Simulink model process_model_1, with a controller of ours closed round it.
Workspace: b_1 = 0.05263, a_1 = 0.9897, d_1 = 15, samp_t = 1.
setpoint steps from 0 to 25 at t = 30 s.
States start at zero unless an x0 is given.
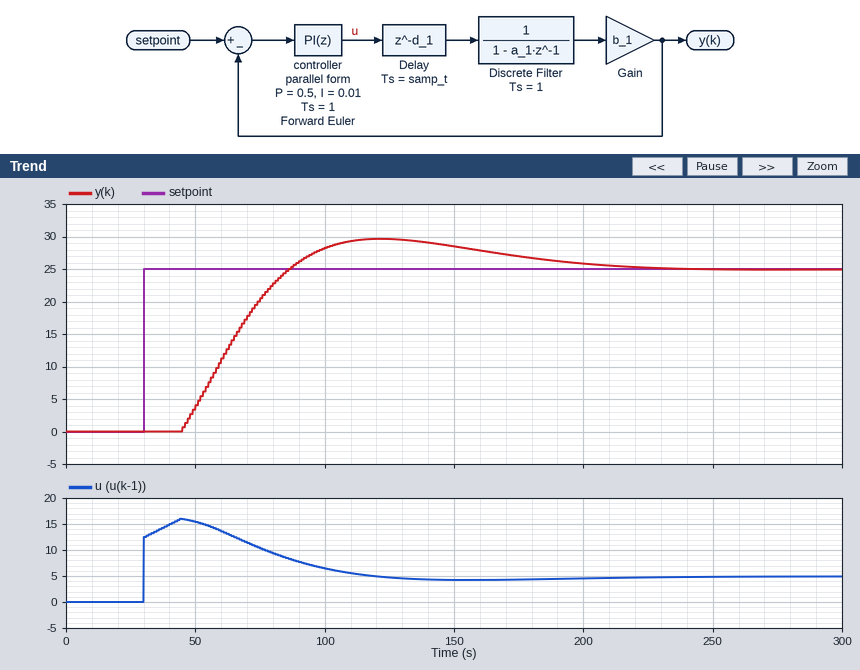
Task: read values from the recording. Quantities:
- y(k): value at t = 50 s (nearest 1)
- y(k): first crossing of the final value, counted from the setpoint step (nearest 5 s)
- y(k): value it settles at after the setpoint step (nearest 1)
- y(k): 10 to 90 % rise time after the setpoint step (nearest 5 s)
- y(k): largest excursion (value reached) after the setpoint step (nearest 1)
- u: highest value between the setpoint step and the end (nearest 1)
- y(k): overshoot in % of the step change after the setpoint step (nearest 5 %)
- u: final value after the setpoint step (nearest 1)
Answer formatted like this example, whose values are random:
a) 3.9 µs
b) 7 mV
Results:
a) 4
b) 55 s
c) 25
d) 30 s
e) 30
f) 16
g) 20 %
h) 5
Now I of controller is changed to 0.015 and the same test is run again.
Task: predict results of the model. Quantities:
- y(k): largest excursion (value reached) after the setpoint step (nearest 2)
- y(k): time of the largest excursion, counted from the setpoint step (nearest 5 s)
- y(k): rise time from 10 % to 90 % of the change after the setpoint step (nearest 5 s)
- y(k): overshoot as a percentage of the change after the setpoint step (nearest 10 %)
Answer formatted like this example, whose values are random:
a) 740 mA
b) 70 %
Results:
a) 34
b) 85 s
c) 25 s
d) 40 %
